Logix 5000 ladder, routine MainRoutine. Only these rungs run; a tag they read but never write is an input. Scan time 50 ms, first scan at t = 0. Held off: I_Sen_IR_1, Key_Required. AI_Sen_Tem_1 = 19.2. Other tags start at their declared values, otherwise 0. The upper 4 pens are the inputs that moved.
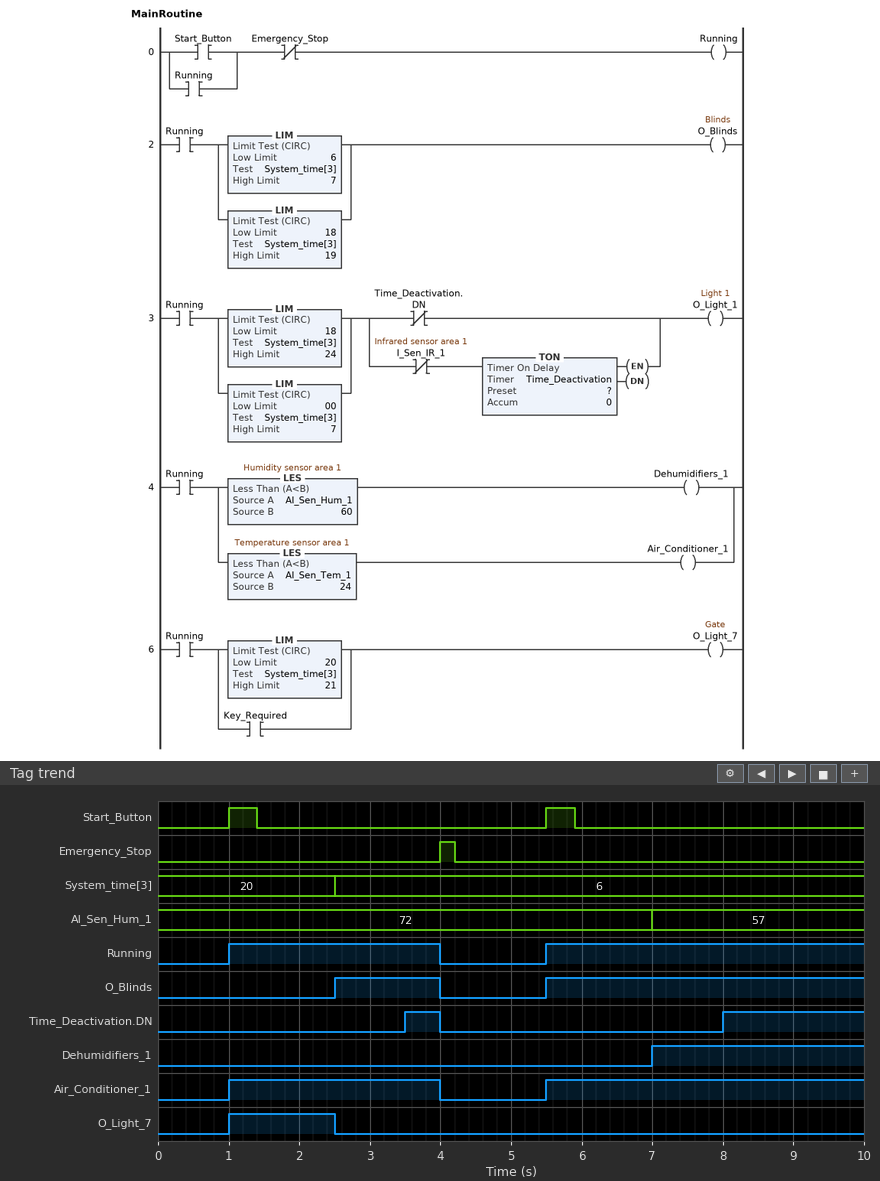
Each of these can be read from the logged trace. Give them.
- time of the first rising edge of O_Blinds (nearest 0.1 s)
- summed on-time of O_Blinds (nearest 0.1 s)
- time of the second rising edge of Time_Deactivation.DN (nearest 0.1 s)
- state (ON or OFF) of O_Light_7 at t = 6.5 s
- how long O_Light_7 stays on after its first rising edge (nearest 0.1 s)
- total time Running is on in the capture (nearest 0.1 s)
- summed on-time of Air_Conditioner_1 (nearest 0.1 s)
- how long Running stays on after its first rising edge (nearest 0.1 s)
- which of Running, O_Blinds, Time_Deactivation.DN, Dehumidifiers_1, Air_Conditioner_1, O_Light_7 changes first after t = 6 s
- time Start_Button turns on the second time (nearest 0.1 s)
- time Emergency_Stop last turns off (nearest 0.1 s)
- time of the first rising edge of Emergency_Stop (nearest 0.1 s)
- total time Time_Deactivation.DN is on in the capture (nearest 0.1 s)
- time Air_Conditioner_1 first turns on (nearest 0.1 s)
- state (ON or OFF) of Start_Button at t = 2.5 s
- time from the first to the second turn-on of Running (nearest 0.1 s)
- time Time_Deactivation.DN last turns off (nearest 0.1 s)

2.5 s
6.0 s
8.0 s
OFF
1.5 s
7.5 s
7.5 s
3.0 s
Dehumidifiers_1
5.5 s
4.2 s
4.0 s
2.5 s
1.0 s
OFF
4.5 s
4.0 s
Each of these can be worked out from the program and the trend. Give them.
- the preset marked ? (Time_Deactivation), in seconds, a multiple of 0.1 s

2.5 s
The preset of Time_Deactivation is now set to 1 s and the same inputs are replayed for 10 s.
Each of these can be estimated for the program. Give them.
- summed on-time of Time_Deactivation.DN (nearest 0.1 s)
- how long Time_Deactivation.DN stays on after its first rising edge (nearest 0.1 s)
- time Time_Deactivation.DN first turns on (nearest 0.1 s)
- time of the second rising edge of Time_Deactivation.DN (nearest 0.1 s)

5.5 s
2.0 s
2.0 s
6.5 s
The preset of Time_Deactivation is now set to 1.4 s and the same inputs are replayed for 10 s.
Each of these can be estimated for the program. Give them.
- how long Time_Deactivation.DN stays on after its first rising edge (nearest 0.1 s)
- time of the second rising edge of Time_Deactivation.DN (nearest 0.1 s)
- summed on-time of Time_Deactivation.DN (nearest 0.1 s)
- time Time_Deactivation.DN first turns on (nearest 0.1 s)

1.6 s
6.9 s
4.7 s
2.4 s
